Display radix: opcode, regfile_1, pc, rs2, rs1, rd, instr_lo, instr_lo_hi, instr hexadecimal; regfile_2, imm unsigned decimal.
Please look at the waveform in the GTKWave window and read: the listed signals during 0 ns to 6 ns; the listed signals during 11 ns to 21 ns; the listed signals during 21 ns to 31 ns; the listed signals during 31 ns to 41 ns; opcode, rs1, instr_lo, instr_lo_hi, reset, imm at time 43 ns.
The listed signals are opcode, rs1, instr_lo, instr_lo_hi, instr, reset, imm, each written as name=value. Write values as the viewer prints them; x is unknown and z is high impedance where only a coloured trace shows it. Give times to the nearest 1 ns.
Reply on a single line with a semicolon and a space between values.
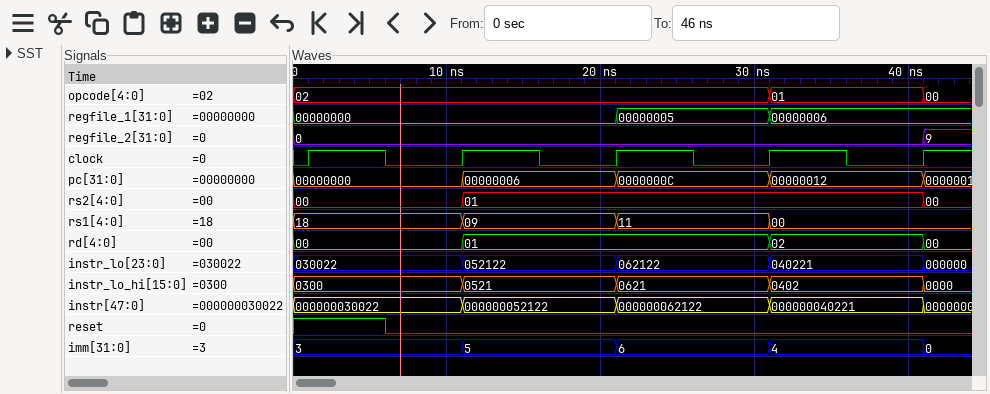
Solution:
opcode=02, rs1=18, instr_lo=030022, instr_lo_hi=0300, instr=000000030022, reset=1, imm=3; opcode=02, rs1=09, instr_lo=052122, instr_lo_hi=0521, instr=000000052122, reset=0, imm=5; opcode=02, rs1=11, instr_lo=062122, instr_lo_hi=0621, instr=000000062122, reset=0, imm=6; opcode=01, rs1=00, instr_lo=040221, instr_lo_hi=0402, instr=000000040221, reset=0, imm=4; opcode=00, rs1=00, instr_lo=000000, instr_lo_hi=0000, reset=0, imm=0
